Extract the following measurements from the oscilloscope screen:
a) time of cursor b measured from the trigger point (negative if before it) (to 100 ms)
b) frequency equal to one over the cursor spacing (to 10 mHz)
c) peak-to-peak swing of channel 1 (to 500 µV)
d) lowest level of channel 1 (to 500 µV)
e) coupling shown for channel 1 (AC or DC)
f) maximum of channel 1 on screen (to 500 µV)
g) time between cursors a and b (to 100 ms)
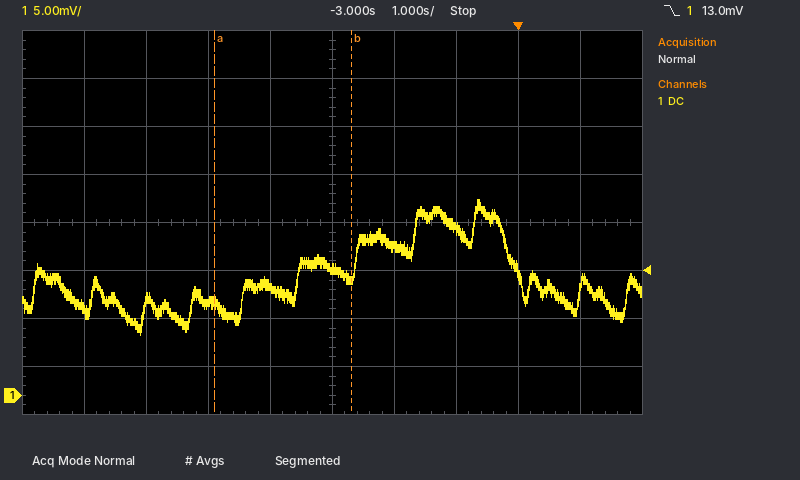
-2.7 s
450 mHz
14.0 mV
6.5 mV
DC
20.5 mV
2.2 s
